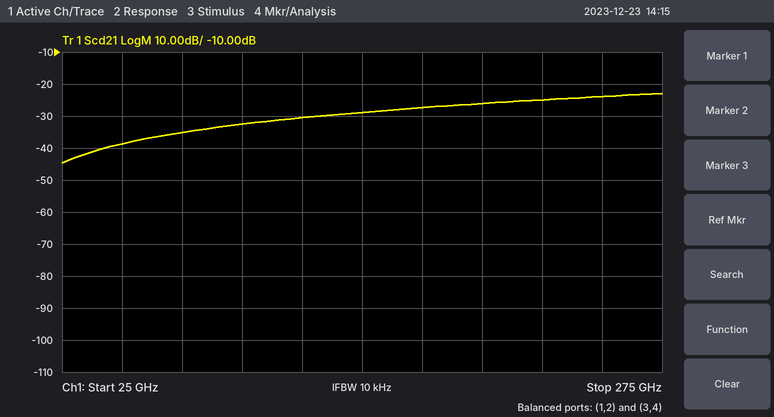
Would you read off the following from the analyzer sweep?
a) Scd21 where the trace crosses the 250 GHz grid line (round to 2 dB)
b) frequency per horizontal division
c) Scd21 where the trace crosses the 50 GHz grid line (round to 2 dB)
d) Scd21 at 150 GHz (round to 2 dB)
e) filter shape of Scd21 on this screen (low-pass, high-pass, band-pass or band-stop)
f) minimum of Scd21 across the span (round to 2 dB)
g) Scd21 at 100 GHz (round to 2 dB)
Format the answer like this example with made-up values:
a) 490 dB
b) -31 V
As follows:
a) -24 dB
b) 25 GHz
c) -38 dB
d) -28 dB
e) high-pass
f) -44 dB
g) -32 dB
